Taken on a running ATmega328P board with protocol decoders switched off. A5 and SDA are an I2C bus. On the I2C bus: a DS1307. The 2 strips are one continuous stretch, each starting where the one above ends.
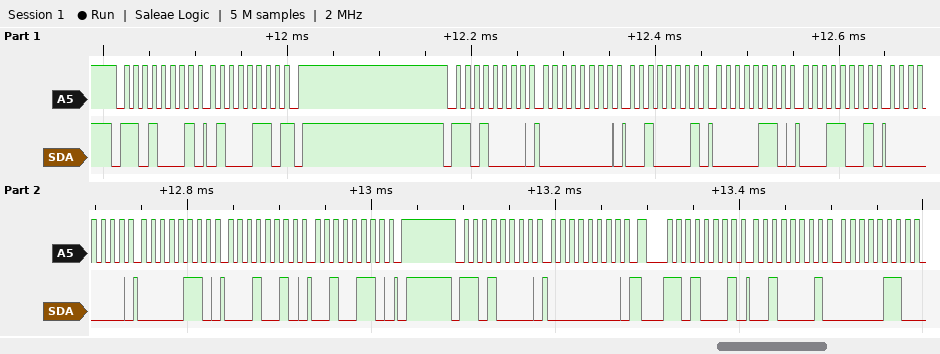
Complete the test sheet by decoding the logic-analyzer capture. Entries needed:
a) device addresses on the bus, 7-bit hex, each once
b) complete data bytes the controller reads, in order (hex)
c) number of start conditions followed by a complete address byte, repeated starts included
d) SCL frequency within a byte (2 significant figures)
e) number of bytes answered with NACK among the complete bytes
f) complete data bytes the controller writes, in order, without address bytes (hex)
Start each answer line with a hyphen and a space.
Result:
- 0x68
- 46 21 06
- 4
- 100 kHz
- 1
- 00 21 06 19 00 06 12 26 00
